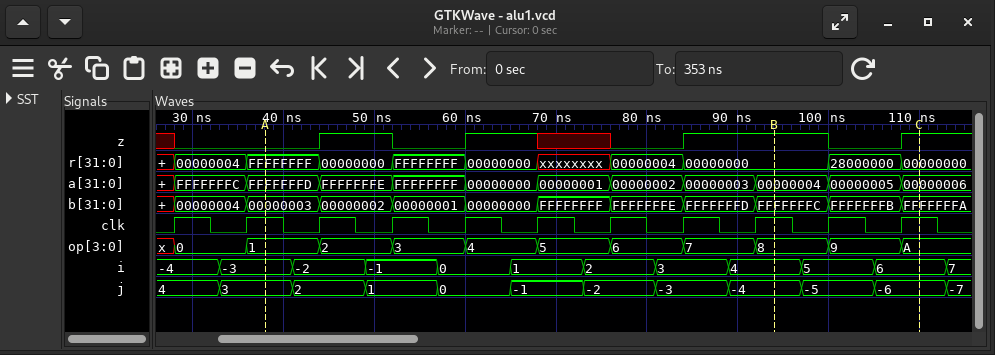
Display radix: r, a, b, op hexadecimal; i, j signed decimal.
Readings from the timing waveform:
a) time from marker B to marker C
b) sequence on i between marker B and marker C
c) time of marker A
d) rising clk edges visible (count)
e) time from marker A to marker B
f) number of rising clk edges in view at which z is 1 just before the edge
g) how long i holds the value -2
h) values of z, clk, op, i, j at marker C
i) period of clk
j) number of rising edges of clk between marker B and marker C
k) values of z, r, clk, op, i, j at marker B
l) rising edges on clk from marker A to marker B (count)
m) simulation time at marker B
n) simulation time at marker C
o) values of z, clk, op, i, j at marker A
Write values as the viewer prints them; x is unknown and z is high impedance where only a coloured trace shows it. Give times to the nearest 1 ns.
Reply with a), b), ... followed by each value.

a) 16 ns
b) 4, 5, 6
c) 38 ns
d) 11
e) 56 ns
f) 4
g) 8 ns
h) z=1, clk=1, op=A, i=6, j=-6
i) 8 ns
j) 2
k) z=1, r=00000000, clk=1, op=8, i=4, j=-4
l) 7
m) 94 ns
n) 110 ns
o) z=0, clk=1, op=1, i=-3, j=3
